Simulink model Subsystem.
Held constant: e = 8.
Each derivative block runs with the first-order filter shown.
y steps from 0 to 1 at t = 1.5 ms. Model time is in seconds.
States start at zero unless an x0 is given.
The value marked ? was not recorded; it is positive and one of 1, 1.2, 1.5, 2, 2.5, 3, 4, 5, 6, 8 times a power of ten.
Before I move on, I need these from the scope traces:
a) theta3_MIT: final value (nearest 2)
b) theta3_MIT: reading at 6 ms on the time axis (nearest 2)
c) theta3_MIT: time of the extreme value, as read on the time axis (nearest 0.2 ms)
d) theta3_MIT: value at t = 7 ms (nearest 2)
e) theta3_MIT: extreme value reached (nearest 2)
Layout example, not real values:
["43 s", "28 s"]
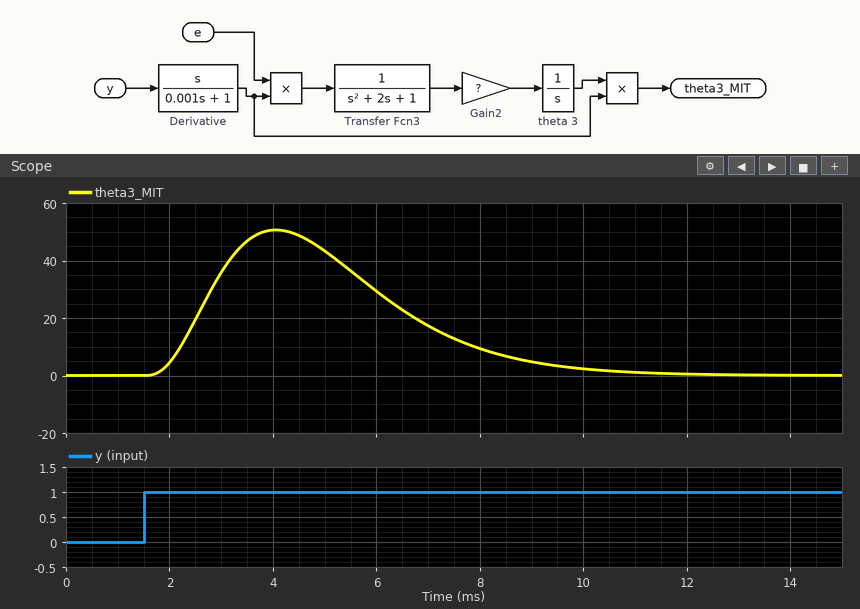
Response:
["0", "30", "4.0 ms", "18", "50"]
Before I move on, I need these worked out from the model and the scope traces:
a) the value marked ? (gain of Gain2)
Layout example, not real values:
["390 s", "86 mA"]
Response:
["50000"]
